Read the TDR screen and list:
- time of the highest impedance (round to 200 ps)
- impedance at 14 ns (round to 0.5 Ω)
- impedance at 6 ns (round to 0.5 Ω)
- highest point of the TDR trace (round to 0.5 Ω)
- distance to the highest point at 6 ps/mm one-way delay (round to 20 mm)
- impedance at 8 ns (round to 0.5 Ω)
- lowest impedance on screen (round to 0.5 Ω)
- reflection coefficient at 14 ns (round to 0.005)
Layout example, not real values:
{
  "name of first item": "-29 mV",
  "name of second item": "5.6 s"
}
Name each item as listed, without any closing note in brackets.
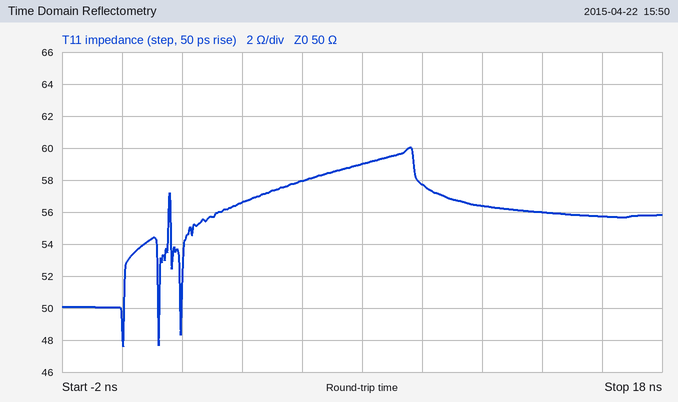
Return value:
{
  "time of the highest impedance": "9.6 ns",
  "impedance at 14 ns": "56.0 Ω",
  "impedance at 6 ns": "58.0 Ω",
  "highest point of the TDR trace": "60.0 Ω",
  "distance to the highest point at 6 ps/mm one-way delay": "800 mm",
  "impedance at 8 ns": "59.0 Ω",
  "lowest impedance on screen": "47.5 Ω",
  "reflection coefficient at 14 ns": "+0.055"
}
